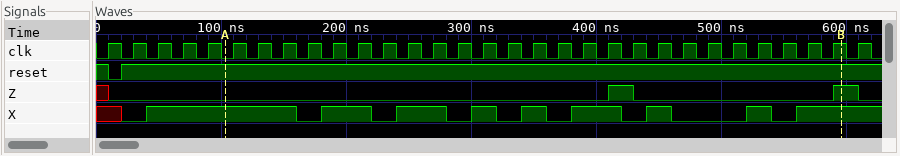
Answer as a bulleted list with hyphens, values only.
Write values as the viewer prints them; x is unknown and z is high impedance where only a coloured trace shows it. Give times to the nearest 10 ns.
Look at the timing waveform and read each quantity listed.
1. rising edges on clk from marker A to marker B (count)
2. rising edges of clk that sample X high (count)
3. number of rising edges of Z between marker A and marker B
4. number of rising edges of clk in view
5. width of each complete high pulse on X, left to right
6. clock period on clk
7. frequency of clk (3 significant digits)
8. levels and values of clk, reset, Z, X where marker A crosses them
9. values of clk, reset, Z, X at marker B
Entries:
- 25
- 19
- 2
- 31
- 120 ns, 40 ns, 40 ns, 20 ns, 20 ns, 40 ns, 20 ns, 20 ns
- 20 ns
- 50.0 MHz
- clk=0, reset=1, Z=0, X=1
- clk=1, reset=1, Z=1, X=1
